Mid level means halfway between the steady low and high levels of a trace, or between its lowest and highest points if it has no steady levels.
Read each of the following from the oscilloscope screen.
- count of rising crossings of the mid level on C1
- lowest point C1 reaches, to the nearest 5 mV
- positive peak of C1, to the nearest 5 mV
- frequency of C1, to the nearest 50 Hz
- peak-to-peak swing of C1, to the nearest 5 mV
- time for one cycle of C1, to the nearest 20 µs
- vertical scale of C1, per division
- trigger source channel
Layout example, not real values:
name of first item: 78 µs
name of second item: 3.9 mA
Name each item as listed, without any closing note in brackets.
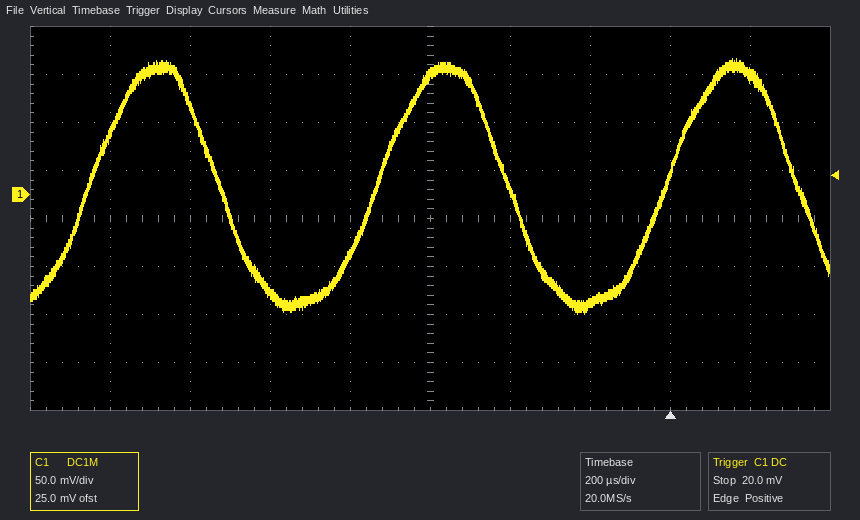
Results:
count of rising crossings of the mid level on C1: 3
lowest point C1 reaches, to the nearest 5 mV: -125 mV
positive peak of C1, to the nearest 5 mV: 140 mV
frequency of C1, to the nearest 50 Hz: 1.40 kHz
peak-to-peak swing of C1, to the nearest 5 mV: 265 mV
time for one cycle of C1, to the nearest 20 µs: 720 µs
vertical scale of C1, per division: 50 mV
trigger source channel: C1
